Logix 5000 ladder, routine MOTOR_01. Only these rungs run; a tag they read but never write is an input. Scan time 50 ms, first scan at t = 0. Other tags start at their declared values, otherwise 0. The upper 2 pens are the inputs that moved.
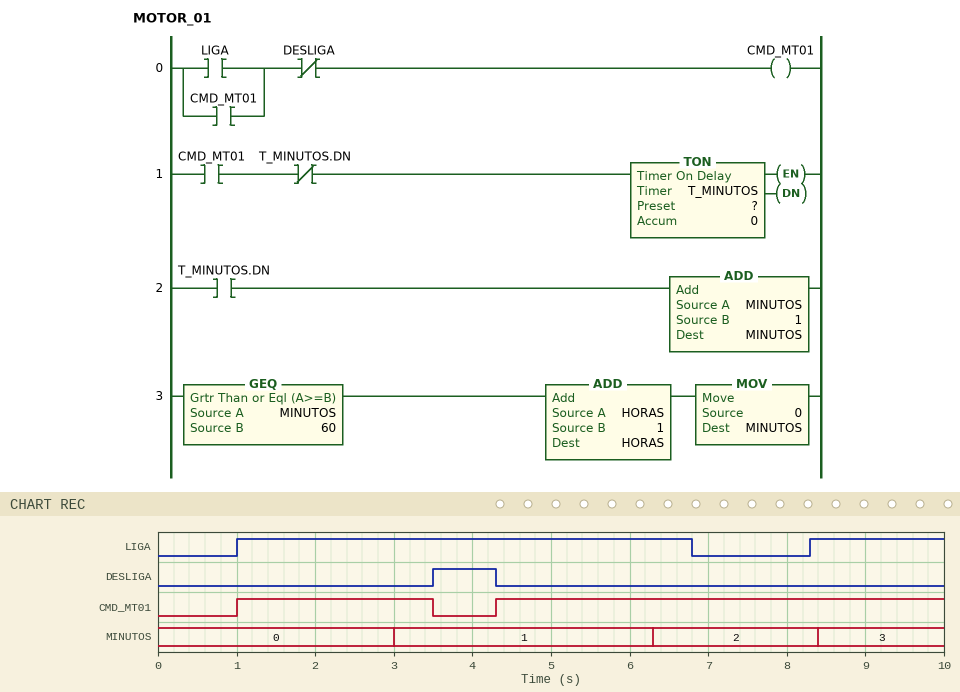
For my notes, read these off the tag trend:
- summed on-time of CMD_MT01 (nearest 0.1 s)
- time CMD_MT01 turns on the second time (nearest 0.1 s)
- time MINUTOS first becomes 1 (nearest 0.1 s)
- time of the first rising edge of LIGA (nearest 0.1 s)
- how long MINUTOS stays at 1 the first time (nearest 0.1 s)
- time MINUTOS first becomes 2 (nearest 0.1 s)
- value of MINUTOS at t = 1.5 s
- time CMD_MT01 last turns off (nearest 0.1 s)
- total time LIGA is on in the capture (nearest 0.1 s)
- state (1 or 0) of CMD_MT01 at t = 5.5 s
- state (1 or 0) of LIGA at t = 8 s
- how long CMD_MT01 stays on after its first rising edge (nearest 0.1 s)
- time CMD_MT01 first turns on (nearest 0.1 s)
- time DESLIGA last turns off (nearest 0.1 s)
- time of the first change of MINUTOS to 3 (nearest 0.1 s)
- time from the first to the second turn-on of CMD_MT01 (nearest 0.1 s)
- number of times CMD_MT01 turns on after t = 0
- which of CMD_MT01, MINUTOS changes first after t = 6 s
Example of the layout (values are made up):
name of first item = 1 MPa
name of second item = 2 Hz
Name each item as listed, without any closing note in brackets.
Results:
summed on-time of CMD_MT01 = 8.2 s
time CMD_MT01 turns on the second time = 4.3 s
time MINUTOS first becomes 1 = 3.0 s
time of the first rising edge of LIGA = 1.0 s
how long MINUTOS stays at 1 the first time = 3.3 s
time MINUTOS first becomes 2 = 6.3 s
value of MINUTOS at t = 1.5 s = 0
time CMD_MT01 last turns off = 3.5 s
total time LIGA is on in the capture = 7.5 s
state (1 or 0) of CMD_MT01 at t = 5.5 s = 1
state (1 or 0) of LIGA at t = 8 s = 0
how long CMD_MT01 stays on after its first rising edge = 2.5 s
time CMD_MT01 first turns on = 1.0 s
time DESLIGA last turns off = 4.3 s
time of the first change of MINUTOS to 3 = 8.4 s
time from the first to the second turn-on of CMD_MT01 = 3.3 s
number of times CMD_MT01 turns on after t = 0 = 2
which of CMD_MT01, MINUTOS changes first after t = 6 s = MINUTOS
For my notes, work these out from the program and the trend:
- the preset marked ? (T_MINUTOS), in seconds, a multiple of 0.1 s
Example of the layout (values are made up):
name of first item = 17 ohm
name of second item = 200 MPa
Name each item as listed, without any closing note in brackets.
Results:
the preset marked ? (T_MINUTOS), in seconds, a multiple of 0.1 s = 2.0 s
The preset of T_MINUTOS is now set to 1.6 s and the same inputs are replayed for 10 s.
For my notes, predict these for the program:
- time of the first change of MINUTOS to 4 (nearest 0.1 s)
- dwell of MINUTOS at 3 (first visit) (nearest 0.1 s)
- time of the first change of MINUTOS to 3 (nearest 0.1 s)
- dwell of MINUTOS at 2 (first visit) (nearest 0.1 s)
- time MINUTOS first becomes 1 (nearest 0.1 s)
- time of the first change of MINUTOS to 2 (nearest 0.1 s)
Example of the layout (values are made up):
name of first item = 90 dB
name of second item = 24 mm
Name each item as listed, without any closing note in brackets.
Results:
time of the first change of MINUTOS to 4 = 9.3 s
dwell of MINUTOS at 3 (first visit) = 1.7 s
time of the first change of MINUTOS to 3 = 7.6 s
dwell of MINUTOS at 2 (first visit) = 1.7 s
time MINUTOS first becomes 1 = 2.6 s
time of the first change of MINUTOS to 2 = 5.9 s
